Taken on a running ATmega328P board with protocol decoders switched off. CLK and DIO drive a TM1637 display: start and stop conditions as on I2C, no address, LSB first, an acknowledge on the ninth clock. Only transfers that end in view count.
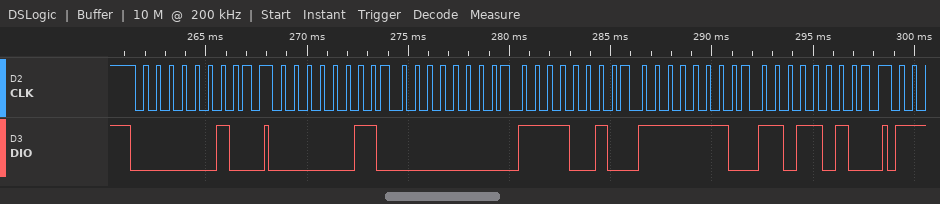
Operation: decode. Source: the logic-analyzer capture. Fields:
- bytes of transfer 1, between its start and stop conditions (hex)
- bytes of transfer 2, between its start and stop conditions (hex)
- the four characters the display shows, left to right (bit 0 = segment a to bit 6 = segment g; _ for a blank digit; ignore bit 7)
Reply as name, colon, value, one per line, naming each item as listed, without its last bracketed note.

bytes of transfer 1, between its start and stop conditions: 40
bytes of transfer 2, between its start and stop conditions: C0 00 4F 7F 5B
the four characters the display shows, left to right: _382
